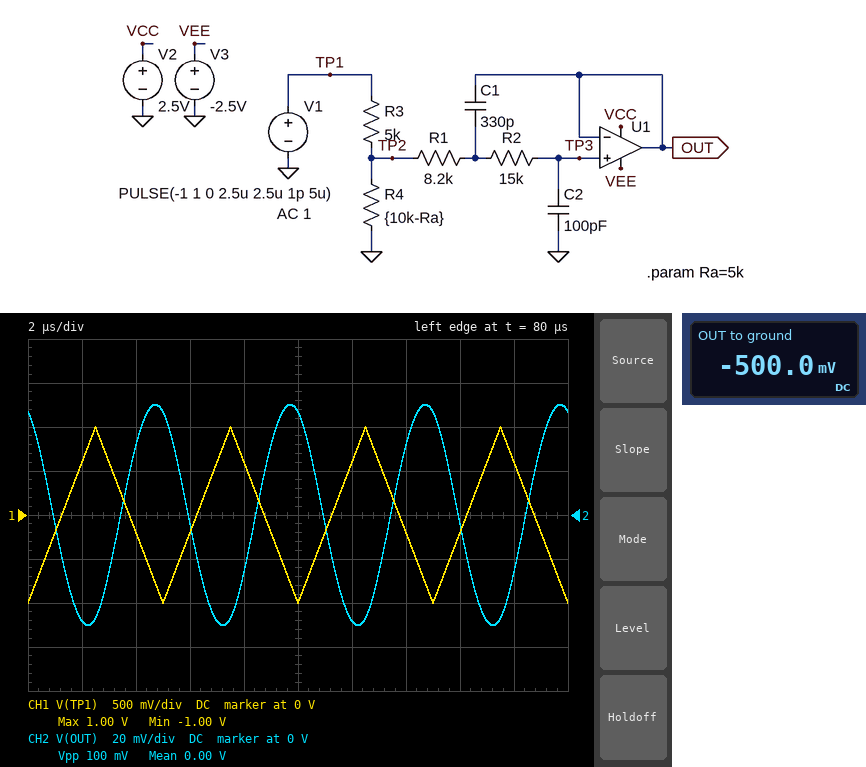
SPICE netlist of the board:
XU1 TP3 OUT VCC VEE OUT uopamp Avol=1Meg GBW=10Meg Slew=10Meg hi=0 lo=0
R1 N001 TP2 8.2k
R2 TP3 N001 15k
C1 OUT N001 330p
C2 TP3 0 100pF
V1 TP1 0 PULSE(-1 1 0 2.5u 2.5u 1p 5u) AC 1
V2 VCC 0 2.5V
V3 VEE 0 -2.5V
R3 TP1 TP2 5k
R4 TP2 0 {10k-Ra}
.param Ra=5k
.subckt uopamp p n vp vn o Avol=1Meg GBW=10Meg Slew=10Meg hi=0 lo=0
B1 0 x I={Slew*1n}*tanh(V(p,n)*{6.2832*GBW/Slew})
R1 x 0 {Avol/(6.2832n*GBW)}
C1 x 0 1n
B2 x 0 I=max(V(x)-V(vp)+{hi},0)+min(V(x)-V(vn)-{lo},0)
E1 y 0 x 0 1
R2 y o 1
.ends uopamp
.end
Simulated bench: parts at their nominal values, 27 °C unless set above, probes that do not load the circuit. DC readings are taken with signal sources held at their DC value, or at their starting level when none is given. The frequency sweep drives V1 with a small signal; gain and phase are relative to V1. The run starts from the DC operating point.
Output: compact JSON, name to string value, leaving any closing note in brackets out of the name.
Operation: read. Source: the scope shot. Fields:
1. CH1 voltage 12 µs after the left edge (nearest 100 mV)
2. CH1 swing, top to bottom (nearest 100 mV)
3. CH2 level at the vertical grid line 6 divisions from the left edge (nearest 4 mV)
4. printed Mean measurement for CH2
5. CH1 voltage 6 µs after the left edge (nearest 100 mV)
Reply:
{"CH1 voltage 12 µs after the left edge": "600 mV", "CH1 swing, top to bottom": "2.0 V", "CH2 level at the vertical grid line 6 divisions from the left edge": "-48 mV", "printed Mean measurement for CH2": "0.00 V", "CH1 voltage 6 µs after the left edge": "-200 mV"}
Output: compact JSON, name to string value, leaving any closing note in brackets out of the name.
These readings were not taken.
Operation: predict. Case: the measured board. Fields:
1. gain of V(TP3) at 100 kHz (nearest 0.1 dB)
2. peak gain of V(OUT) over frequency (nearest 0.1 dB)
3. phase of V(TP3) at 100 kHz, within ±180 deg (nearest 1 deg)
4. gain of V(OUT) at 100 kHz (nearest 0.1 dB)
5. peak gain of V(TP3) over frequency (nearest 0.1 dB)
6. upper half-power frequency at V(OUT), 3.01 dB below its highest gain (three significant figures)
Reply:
{"gain of V(TP3) at 100 kHz": "-11.9 dB", "peak gain of V(OUT) over frequency": "-5.3 dB", "phase of V(TP3) at 100 kHz, within ±180 deg": "-125 deg", "gain of V(OUT) at 100 kHz": "-11.9 dB", "peak gain of V(TP3) over frequency": "-5.3 dB", "upper half-power frequency at V(OUT), 3.01 dB below its highest gain": "78.6 kHz"}
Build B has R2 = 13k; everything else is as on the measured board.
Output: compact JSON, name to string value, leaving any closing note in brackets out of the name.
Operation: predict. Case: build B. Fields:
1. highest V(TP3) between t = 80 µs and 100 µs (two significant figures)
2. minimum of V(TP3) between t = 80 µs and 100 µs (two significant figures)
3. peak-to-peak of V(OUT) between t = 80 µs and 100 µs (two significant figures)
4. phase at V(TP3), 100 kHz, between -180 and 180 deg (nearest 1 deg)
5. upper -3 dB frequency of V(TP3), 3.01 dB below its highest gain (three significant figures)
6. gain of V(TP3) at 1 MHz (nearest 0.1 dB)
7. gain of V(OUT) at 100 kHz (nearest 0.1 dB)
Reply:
{"highest V(TP3) between t = 80 µs and 100 µs": "58 mV", "minimum of V(TP3) between t = 80 µs and 100 µs": "-58 mV", "peak-to-peak of V(OUT) between t = 80 µs and 100 µs": "120 mV", "phase at V(TP3), 100 kHz, between -180 and 180 deg": "-119 deg", "upper -3 dB frequency of V(TP3), 3.01 dB below its highest gain": "84.6 kHz", "gain of V(TP3) at 1 MHz": "-51.3 dB", "gain of V(OUT) at 100 kHz": "-10.7 dB"}
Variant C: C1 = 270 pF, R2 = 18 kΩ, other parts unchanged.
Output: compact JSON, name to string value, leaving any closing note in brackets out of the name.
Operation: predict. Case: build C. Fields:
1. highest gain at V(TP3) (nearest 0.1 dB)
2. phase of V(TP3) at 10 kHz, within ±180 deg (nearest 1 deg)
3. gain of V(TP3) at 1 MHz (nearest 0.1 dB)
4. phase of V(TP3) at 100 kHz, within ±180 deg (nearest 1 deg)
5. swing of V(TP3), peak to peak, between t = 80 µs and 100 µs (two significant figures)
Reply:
{"highest gain at V(TP3)": "-5.8 dB", "phase of V(TP3) at 10 kHz, within ±180 deg": "-10 deg", "gain of V(TP3) at 1 MHz": "-52.3 dB", "phase of V(TP3) at 100 kHz, within ±180 deg": "-121 deg", "swing of V(TP3), peak to peak, between t = 80 µs and 100 µs": "100 mV"}
